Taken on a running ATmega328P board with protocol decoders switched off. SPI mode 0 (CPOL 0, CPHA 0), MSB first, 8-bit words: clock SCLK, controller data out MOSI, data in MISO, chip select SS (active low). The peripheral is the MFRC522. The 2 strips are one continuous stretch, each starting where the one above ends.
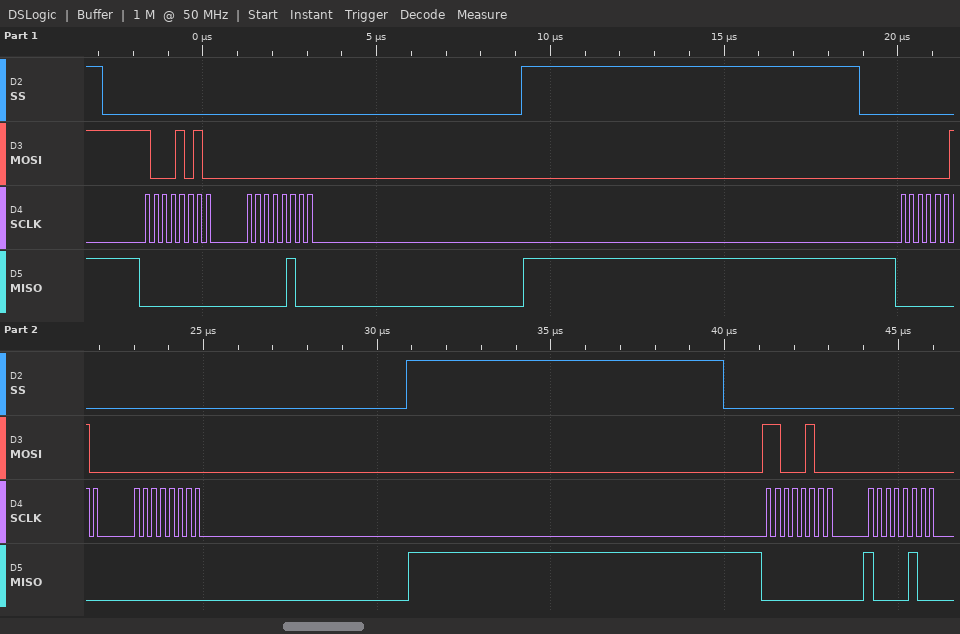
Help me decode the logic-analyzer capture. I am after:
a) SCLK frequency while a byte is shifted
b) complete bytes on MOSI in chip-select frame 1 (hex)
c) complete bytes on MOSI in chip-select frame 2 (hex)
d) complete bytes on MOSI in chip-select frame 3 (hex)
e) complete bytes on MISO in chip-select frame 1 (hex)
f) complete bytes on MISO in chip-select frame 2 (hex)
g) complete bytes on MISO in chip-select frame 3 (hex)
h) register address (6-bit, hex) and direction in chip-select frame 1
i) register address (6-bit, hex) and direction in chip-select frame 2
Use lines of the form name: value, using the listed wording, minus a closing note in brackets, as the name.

SCLK frequency while a byte is shifted: 4 MHz
complete bytes on MOSI in chip-select frame 1: 8A 00
complete bytes on MOSI in chip-select frame 2: 02 00
complete bytes on MOSI in chip-select frame 3: C4 00
complete bytes on MISO in chip-select frame 1: 00 04
complete bytes on MISO in chip-select frame 2: 00 00
complete bytes on MISO in chip-select frame 3: 00 84
register address (6-bit, hex) and direction in chip-select frame 1: 0x05 read
register address (6-bit, hex) and direction in chip-select frame 2: 0x01 write
